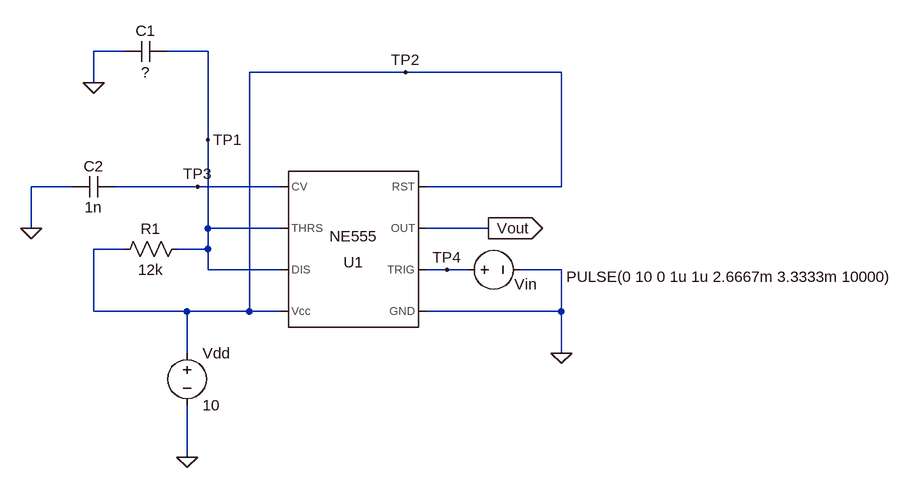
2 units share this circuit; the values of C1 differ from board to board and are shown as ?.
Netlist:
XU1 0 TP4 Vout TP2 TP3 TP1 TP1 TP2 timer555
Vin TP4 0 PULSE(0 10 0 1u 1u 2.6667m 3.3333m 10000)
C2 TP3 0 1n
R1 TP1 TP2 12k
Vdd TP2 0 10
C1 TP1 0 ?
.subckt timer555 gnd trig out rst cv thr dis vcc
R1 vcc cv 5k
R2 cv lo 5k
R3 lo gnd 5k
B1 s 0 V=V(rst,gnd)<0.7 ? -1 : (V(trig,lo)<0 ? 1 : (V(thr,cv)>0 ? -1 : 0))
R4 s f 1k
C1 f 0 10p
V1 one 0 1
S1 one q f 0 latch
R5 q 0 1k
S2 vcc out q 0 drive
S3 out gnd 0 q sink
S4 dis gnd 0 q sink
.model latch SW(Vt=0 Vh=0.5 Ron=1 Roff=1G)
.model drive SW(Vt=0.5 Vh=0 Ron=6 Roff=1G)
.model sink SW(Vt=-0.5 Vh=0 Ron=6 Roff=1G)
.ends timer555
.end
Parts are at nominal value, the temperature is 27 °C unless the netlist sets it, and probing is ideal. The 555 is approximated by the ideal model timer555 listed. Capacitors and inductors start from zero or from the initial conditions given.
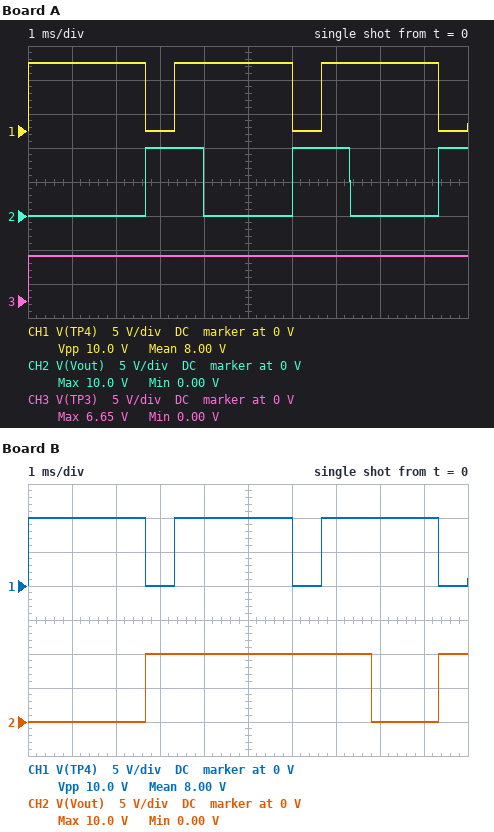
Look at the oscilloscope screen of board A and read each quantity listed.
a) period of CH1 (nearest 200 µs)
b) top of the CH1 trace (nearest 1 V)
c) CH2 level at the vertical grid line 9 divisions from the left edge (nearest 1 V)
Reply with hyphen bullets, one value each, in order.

- 3.4 ms
- 10 V
- 0 V
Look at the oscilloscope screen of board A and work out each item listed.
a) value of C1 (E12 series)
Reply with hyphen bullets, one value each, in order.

- 100 nF
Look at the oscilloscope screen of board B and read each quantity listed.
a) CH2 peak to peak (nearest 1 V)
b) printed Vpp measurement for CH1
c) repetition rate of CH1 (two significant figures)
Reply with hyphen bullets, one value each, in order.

- 10 V
- 10.0 V
- 300 Hz
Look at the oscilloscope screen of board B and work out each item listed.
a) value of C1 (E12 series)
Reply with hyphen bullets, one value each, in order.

- 390 nF
